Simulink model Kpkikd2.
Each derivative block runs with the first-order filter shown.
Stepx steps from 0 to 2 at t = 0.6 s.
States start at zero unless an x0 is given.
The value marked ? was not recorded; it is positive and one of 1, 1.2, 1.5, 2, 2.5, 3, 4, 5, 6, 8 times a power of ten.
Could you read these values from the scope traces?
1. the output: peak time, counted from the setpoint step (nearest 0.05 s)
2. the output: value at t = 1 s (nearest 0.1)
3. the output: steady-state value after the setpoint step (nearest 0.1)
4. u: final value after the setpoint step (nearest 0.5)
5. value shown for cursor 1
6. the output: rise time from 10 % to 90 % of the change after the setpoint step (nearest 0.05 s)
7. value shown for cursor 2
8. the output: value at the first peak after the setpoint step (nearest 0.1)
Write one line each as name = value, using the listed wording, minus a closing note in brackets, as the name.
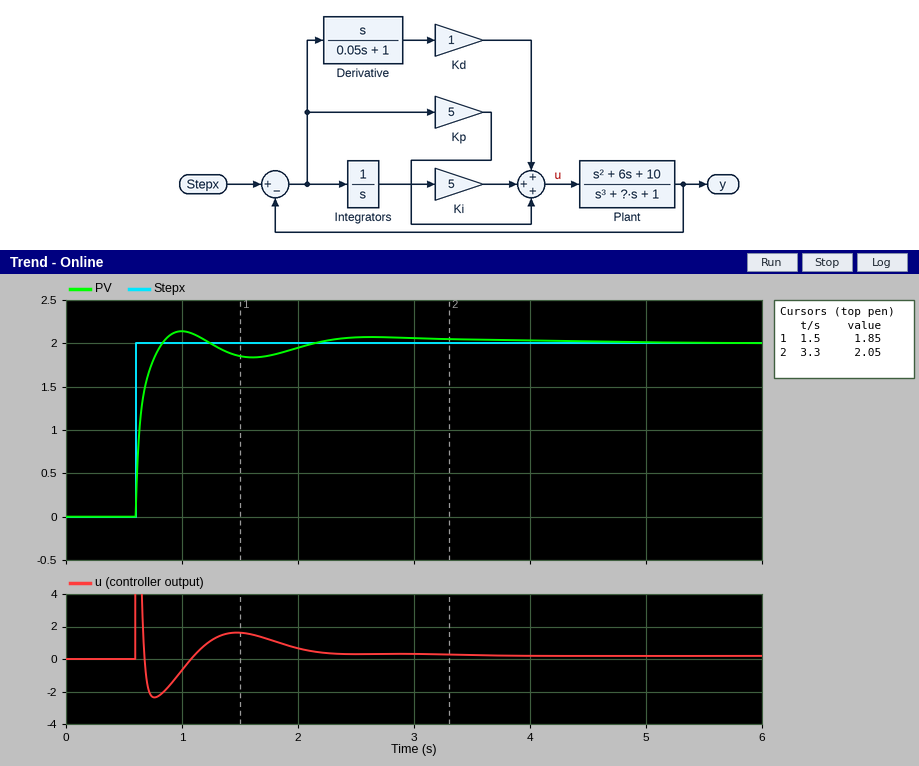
the output: peak time, counted from the setpoint step = 0.40 s
the output: value at t = 1 s = 2.1
the output: steady-state value after the setpoint step = 2.0
u: final value after the setpoint step = 0.0
value shown for cursor 1 = 1.85
the output: rise time from 10 % to 90 % of the change after the setpoint step = 0.15 s
value shown for cursor 2 = 2.05
the output: value at the first peak after the setpoint step = 2.1
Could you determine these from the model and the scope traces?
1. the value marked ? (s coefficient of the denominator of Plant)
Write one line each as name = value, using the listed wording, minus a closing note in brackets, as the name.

the value marked ? = 8
